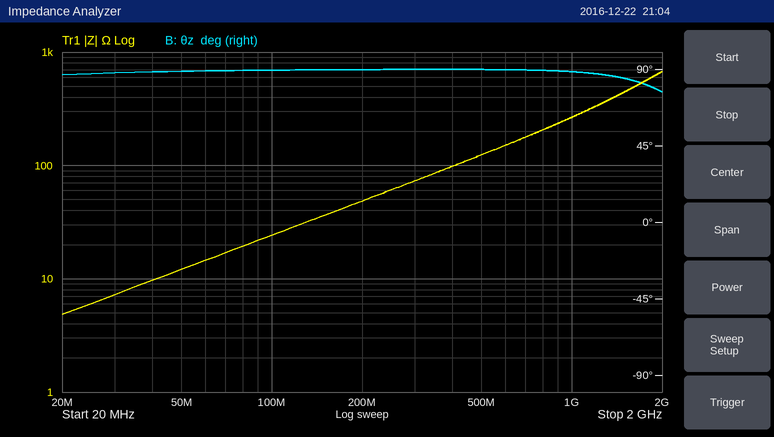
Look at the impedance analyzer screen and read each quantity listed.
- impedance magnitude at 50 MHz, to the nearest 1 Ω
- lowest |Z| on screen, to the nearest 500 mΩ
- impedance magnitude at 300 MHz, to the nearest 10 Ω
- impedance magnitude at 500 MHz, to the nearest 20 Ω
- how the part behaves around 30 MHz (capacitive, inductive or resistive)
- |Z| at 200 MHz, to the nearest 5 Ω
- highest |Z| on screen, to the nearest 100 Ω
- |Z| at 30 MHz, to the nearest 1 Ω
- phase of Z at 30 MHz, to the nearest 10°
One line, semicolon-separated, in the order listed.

12 Ω; 5.0 Ω; 70 Ω; 120 Ω; inductive; 50 Ω; 700 Ω; 7 Ω; 90°
